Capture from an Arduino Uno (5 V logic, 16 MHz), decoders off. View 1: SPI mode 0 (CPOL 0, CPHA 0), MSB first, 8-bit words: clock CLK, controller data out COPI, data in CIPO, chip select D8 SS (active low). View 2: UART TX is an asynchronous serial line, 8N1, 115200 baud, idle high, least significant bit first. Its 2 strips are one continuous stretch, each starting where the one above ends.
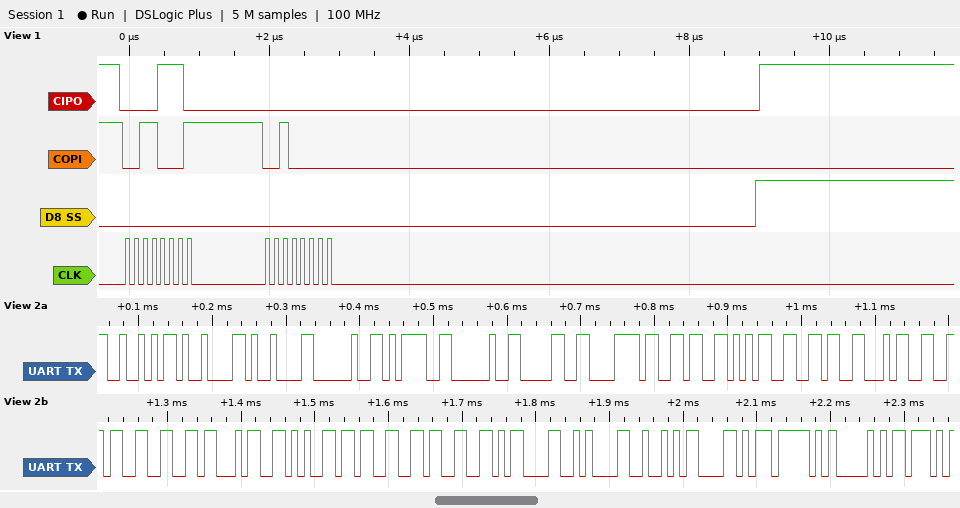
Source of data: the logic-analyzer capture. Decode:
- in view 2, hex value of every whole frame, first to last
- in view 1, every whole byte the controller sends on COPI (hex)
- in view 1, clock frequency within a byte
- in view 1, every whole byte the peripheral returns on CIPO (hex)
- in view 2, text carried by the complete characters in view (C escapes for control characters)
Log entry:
0x52 0x09 0x09 0x20 0x3D 0x20 0x30 0x78 0x36 0x35 0x36 0x34 0x36 0x66 0x34 0x65 0x33 0x33 0x0D 0x0A 0x52 0x58 0x5F 0x50
31 20
8 MHz
0E 00
"R\t\t = 0x65646f4e33\r\nRX_P"
